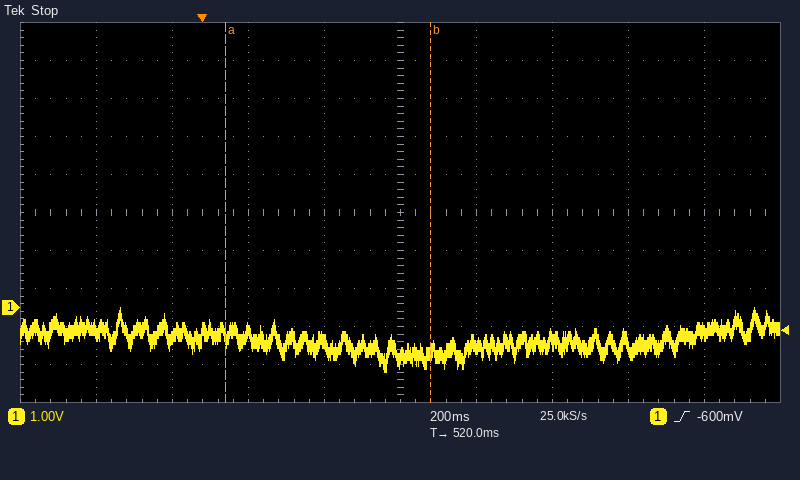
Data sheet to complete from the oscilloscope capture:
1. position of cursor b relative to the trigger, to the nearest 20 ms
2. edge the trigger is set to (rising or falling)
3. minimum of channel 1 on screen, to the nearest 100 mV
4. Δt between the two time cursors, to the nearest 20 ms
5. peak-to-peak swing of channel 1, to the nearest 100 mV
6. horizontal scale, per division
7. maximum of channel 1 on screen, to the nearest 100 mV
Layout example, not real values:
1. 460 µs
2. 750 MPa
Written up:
1. +600 ms
2. rising
3. -1.7 V
4. 540 ms
5. 1.7 V
6. 200 ms
7. 0.0 V
